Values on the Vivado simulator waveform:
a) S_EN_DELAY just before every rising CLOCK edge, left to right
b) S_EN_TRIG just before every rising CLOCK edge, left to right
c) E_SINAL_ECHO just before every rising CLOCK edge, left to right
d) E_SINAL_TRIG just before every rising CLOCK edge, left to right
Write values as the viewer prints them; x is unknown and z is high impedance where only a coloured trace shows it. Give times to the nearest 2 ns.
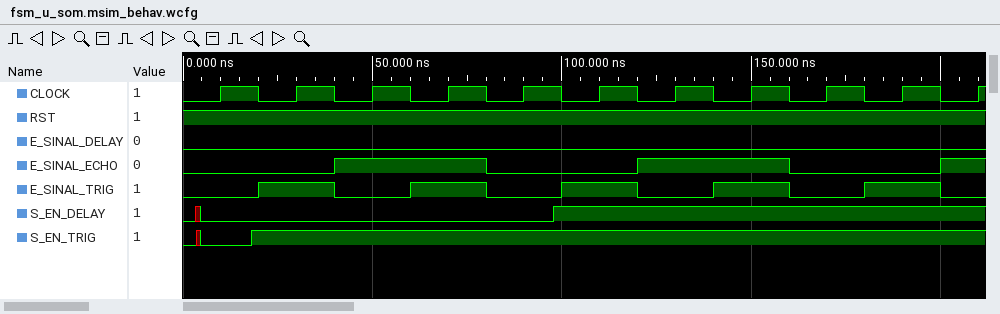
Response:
0 0 0 0 0 1 1 1 1 1 1
0 1 1 1 1 1 1 1 1 1 1
0 0 1 1 0 0 1 1 0 0 1
0 1 0 1 0 1 0 1 0 1 0
